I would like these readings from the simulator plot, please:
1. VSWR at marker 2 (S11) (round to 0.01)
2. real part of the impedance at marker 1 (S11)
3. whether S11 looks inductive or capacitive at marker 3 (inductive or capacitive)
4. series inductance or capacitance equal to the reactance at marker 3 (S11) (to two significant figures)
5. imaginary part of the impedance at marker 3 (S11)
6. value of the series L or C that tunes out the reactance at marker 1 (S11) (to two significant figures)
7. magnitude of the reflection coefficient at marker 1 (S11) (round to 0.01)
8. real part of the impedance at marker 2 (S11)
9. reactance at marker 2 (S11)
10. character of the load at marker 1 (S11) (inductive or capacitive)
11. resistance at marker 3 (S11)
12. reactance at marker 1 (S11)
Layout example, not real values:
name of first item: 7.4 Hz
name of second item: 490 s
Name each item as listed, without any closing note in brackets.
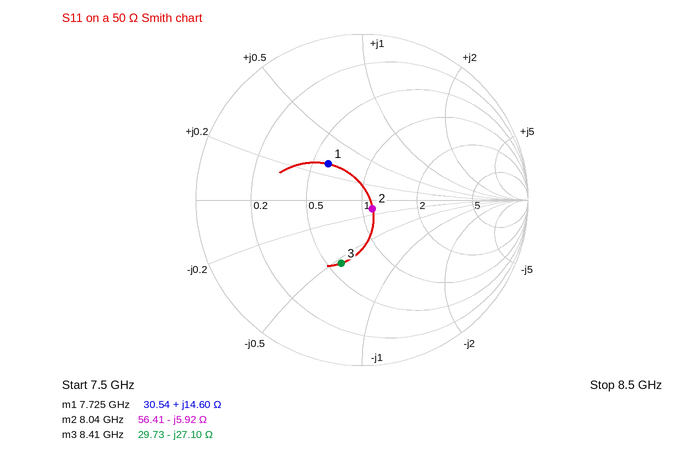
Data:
VSWR at marker 2 (S11): 1.18
real part of the impedance at marker 1: 30.54 Ω
whether S11 looks inductive or capacitive at marker 3: capacitive
series inductance or capacitance equal to the reactance at marker 3 (S11): 700 fF
imaginary part of the impedance at marker 3: -27.10 Ω
value of the series L or C that tunes out the reactance at marker 1 (S11): 1.4 pF
magnitude of the reflection coefficient at marker 1 (S11): 0.30
real part of the impedance at marker 2: 56.41 Ω
reactance at marker 2: -5.92 Ω
character of the load at marker 1 (S11): inductive
resistance at marker 3: 29.73 Ω
reactance at marker 1: +14.60 Ω
